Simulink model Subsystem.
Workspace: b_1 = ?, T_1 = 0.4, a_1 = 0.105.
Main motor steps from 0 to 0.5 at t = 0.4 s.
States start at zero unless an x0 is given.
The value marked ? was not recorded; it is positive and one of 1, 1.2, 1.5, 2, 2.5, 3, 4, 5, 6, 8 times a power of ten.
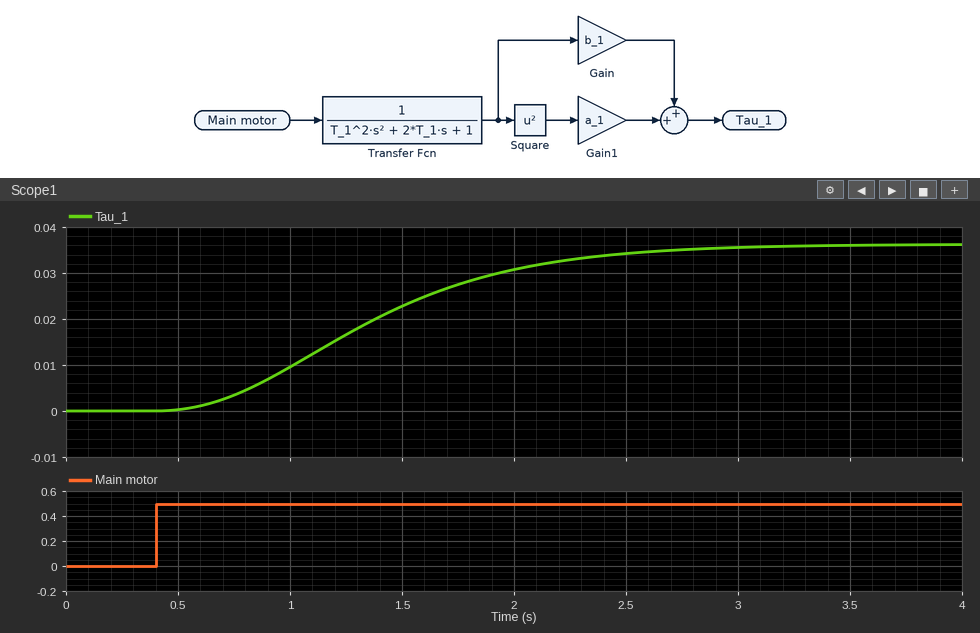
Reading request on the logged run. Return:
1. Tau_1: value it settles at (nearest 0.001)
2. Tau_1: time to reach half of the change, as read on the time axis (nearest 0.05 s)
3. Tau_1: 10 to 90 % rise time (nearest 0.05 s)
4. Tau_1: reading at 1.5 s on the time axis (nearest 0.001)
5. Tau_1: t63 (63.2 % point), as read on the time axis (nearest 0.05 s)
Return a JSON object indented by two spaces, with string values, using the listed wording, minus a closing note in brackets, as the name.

{
  "Tau_1: value it settles at": "0.036",
  "Tau_1: time to reach half of the change, as read on the time axis": "1.30 s",
  "Tau_1: 10 to 90 % rise time": "1.45 s",
  "Tau_1: reading at 1.5 s on the time axis": "0.023",
  "Tau_1: t63 (63.2 % point), as read on the time axis": "1.50 s"
}
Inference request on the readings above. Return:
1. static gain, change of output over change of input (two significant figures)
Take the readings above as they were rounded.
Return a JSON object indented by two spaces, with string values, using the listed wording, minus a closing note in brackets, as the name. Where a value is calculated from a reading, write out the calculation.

{
  "static gain, change of output over change of input": "(0.036 - 0) / (0.5 - 0) = 0.072"
}
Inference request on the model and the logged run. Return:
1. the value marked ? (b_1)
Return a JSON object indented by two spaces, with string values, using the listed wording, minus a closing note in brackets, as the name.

{
  "the value marked ?": "0.02"
}
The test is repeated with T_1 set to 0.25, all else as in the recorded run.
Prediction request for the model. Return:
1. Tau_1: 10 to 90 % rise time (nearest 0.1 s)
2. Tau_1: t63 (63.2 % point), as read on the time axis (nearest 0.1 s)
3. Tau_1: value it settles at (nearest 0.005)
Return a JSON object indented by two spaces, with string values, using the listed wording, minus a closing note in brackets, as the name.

{
  "Tau_1: 10 to 90 % rise time": "0.9 s",
  "Tau_1: t63 (63.2 % point), as read on the time axis": "1.1 s",
  "Tau_1: value it settles at": "0.035"
}
